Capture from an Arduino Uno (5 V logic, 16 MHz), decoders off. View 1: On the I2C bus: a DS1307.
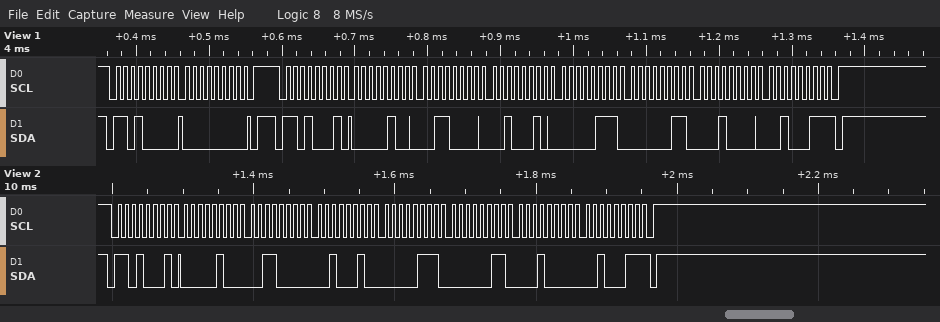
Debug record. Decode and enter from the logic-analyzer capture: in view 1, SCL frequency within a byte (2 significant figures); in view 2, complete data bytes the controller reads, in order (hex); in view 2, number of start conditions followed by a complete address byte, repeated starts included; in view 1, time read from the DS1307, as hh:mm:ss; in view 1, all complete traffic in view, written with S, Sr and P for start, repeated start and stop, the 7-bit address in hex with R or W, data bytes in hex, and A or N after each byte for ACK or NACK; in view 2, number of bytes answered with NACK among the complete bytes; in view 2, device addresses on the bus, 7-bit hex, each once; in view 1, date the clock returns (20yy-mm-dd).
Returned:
100 kHz
04 30 22 07 03 10 23
1
22:30:04
S 68W A 00 A P S 68R A 04 A 30 A 22 A 07 A 03 A 10 A 23 N P
1
0x68
2023-10-03
